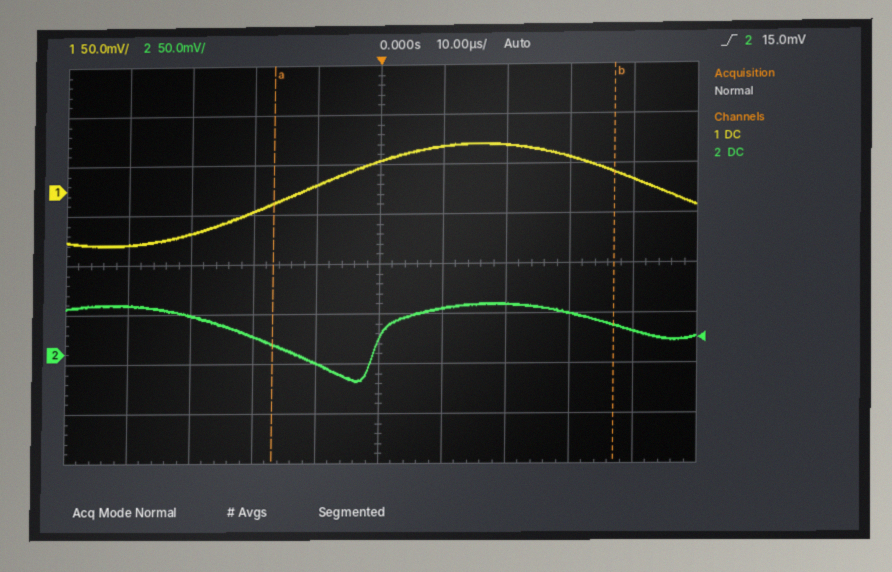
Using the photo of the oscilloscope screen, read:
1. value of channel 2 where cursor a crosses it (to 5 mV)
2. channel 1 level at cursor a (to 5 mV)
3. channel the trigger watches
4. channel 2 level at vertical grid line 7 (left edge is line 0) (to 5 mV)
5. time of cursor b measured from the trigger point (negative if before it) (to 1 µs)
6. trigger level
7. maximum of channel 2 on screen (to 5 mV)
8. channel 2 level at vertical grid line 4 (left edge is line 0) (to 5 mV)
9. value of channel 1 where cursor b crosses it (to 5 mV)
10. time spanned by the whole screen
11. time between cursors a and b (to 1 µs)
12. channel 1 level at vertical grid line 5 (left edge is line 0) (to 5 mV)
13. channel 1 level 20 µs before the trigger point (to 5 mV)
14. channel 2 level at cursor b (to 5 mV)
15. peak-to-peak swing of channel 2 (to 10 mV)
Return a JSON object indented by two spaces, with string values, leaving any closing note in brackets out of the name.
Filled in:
{
  "value of channel 2 where cursor a crosses it": "10 mV",
  "channel 1 level at cursor a": "-15 mV",
  "channel the trigger watches": "channel 2",
  "channel 2 level at vertical grid line 7 (left edge is line 0)": "50 mV",
  "time of cursor b measured from the trigger point (negative if before it)": "+37 µs",
  "trigger level": "15.0 mV",
  "maximum of channel 2 on screen": "50 mV",
  "channel 2 level at vertical grid line 4 (left edge is line 0)": "-10 mV",
  "value of channel 1 where cursor b crosses it": "15 mV",
  "time spanned by the whole screen": "100 µs",
  "time between cursors a and b": "54 µs",
  "channel 1 level at vertical grid line 5 (left edge is line 0)": "30 mV",
  "channel 1 level 20 µs before the trigger point": "-20 mV",
  "channel 2 level at cursor b": "30 mV",
  "peak-to-peak swing of channel 2": "80 mV"
}
